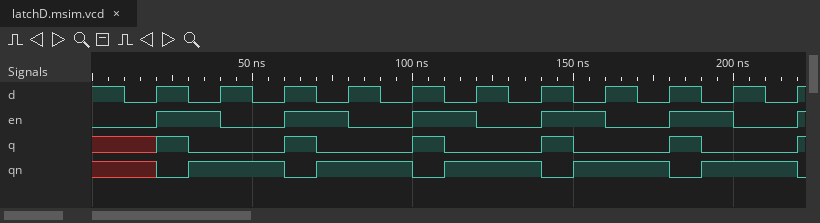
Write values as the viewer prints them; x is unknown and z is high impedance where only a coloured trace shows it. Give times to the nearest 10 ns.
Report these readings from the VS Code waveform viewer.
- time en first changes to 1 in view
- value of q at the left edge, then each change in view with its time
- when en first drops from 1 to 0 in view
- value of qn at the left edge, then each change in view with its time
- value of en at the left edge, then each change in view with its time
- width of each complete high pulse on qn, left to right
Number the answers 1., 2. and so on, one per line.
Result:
1. 20 ns
2. x, 1 at 20 ns, 0 at 30 ns, 1 at 60 ns, 0 at 70 ns, 1 at 100 ns, 0 at 110 ns, 1 at 140 ns, 0 at 150 ns, 1 at 180 ns, 0 at 190 ns, 1 at 220 ns
3. 40 ns
4. x, 0 at 20 ns, 1 at 30 ns, 0 at 60 ns, 1 at 70 ns, 0 at 100 ns, 1 at 110 ns, 0 at 140 ns, 1 at 150 ns, 0 at 180 ns, 1 at 190 ns, 0 at 220 ns
5. 0, 1 at 20 ns, 0 at 40 ns, 1 at 60 ns, 0 at 80 ns, 1 at 100 ns, 0 at 120 ns, 1 at 140 ns, 0 at 160 ns, 1 at 180 ns, 0 at 200 ns, 1 at 220 ns
6. 30 ns, 30 ns, 30 ns, 30 ns, 30 ns
